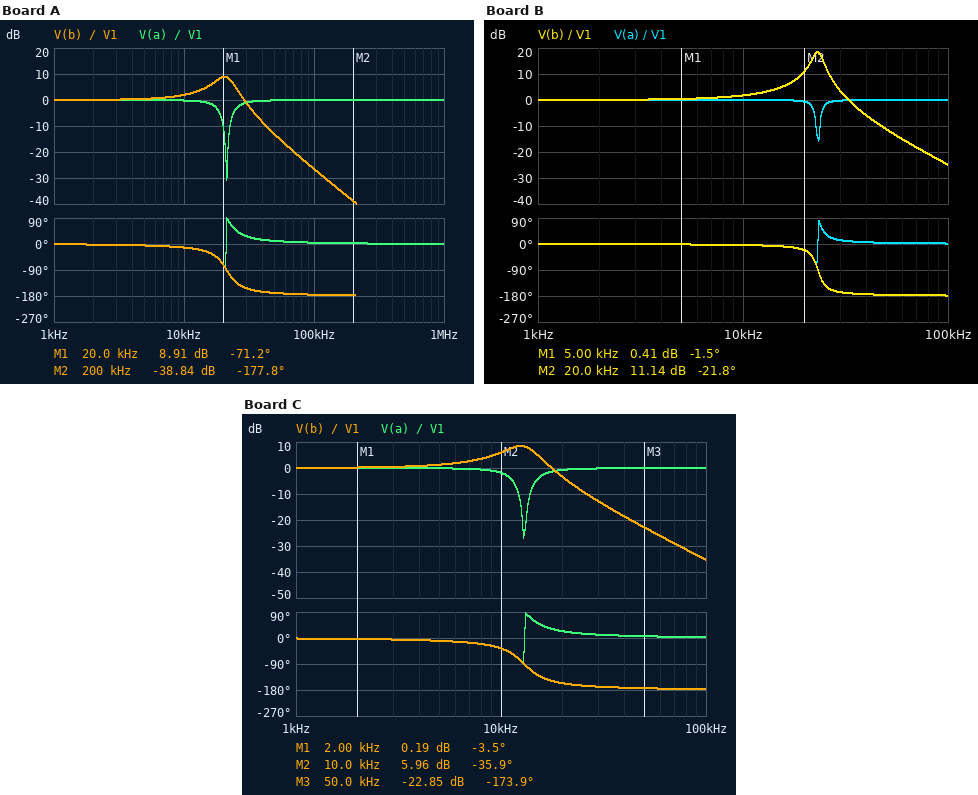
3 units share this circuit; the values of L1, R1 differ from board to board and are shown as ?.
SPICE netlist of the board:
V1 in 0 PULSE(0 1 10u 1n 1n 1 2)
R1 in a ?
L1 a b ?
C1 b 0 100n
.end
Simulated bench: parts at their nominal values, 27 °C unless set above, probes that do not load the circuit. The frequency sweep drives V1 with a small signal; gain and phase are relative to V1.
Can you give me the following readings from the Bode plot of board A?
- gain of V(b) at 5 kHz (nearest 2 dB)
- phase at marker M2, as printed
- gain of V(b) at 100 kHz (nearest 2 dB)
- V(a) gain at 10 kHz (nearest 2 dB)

0 dB
-177.8 deg
-26 dB
0 dB
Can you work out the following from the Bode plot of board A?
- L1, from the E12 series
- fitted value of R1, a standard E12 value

560 µH
27 Ω
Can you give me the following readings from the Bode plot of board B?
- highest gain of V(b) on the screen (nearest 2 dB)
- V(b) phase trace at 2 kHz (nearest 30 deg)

18 dB
0 deg
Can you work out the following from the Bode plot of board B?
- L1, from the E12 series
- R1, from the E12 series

470 µH
8.2 Ω
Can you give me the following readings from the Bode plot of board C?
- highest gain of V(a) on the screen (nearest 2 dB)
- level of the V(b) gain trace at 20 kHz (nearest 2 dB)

0 dB
-4 dB
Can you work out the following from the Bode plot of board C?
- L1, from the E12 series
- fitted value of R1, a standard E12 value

1.5 mH
47 Ω
